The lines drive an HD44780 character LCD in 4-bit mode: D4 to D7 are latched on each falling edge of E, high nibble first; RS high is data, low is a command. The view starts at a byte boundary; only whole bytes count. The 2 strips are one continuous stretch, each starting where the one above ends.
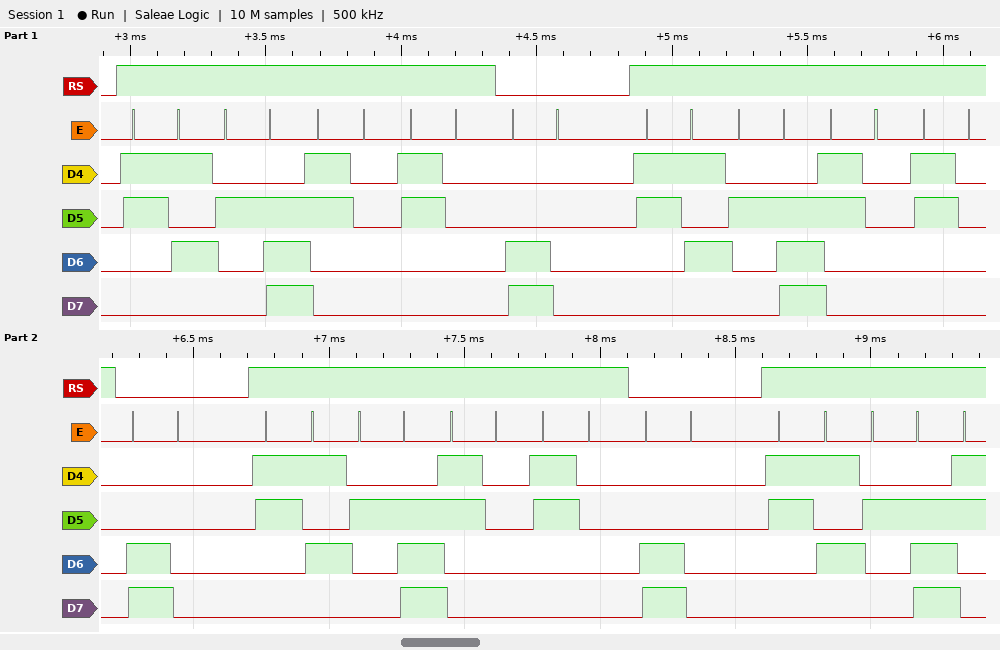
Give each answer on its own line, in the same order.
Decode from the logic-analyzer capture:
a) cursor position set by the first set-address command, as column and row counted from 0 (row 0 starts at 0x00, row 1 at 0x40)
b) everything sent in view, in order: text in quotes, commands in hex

column 0, row 1
"5.00" 0xC0 "5.00" 0xC0 "5.00" 0xC0 "5."
